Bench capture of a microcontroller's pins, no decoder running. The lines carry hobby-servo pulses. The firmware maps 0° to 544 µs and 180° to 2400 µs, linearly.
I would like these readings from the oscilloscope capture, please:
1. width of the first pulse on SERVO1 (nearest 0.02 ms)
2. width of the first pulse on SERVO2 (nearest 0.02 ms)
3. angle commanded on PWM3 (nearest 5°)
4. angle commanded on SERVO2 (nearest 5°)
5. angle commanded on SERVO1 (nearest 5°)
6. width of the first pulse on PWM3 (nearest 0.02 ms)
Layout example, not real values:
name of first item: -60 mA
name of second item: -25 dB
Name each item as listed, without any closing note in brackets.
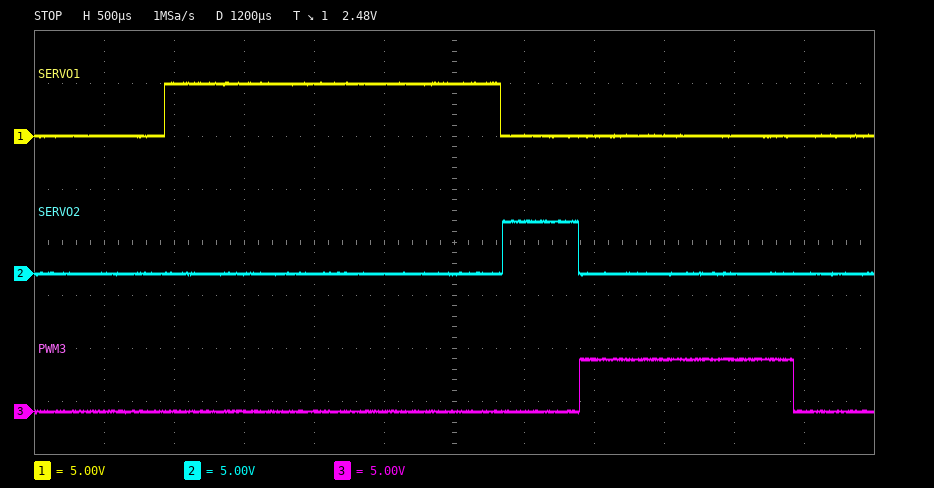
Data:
width of the first pulse on SERVO1: 2.40 ms
width of the first pulse on SERVO2: 0.54 ms
angle commanded on PWM3: 95°
angle commanded on SERVO2: 0°
angle commanded on SERVO1: 180°
width of the first pulse on PWM3: 1.52 ms
